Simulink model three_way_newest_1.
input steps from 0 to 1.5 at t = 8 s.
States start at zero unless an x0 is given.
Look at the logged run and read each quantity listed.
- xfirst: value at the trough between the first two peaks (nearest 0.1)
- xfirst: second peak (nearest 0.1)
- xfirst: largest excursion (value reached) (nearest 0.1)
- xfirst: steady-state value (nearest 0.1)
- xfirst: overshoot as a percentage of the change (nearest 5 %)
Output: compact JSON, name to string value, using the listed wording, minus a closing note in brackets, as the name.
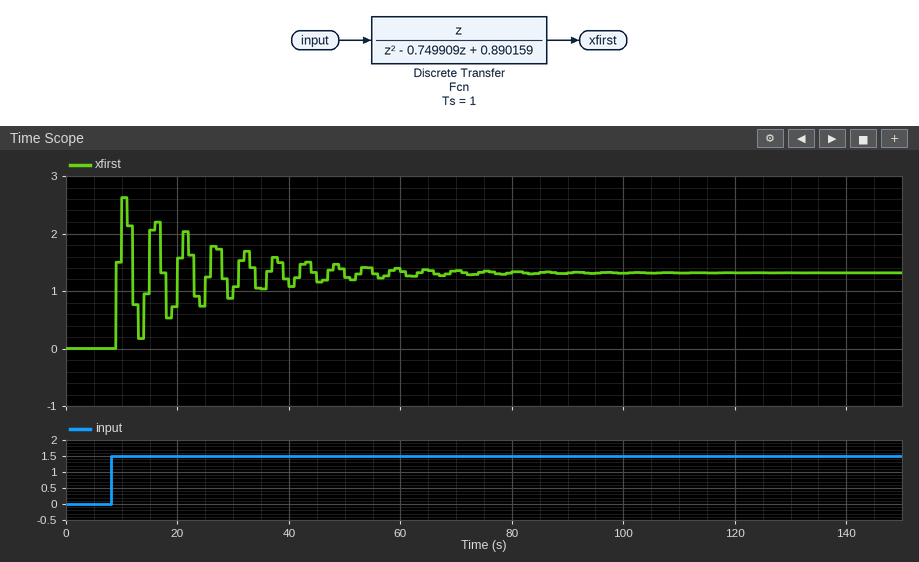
{"xfirst: value at the trough between the first two peaks": "0.2", "xfirst: second peak": "2.2", "xfirst: largest excursion (value reached)": "2.6", "xfirst: steady-state value": "1.3", "xfirst: overshoot as a percentage of the change": "100 %"}
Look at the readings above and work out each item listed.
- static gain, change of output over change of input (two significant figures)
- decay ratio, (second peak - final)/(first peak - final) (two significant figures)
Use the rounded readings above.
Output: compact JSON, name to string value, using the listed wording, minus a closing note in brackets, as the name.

{"static gain, change of output over change of input": "0.87", "decay ratio, (second peak - final)/(first peak - final)": "0.69"}
